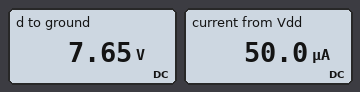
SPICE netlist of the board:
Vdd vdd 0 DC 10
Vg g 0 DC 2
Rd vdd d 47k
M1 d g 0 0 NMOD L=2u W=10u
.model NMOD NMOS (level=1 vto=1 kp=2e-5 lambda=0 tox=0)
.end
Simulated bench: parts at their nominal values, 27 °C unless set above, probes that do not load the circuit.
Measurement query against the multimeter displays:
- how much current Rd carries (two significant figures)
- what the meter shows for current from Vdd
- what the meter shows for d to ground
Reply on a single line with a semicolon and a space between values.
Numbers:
50 µA; 50.0 µA; 7.65 V
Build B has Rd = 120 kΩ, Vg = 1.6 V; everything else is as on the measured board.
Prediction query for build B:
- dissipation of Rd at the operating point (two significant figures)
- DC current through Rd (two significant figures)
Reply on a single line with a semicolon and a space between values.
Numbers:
39 µW; 18 µA
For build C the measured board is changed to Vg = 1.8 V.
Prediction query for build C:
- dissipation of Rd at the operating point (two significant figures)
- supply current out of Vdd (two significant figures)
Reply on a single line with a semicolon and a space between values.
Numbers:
48 µW; 32 µA
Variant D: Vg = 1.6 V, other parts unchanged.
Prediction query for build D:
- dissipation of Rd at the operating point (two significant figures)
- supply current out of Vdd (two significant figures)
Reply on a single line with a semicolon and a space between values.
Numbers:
15 µW; 18 µA
